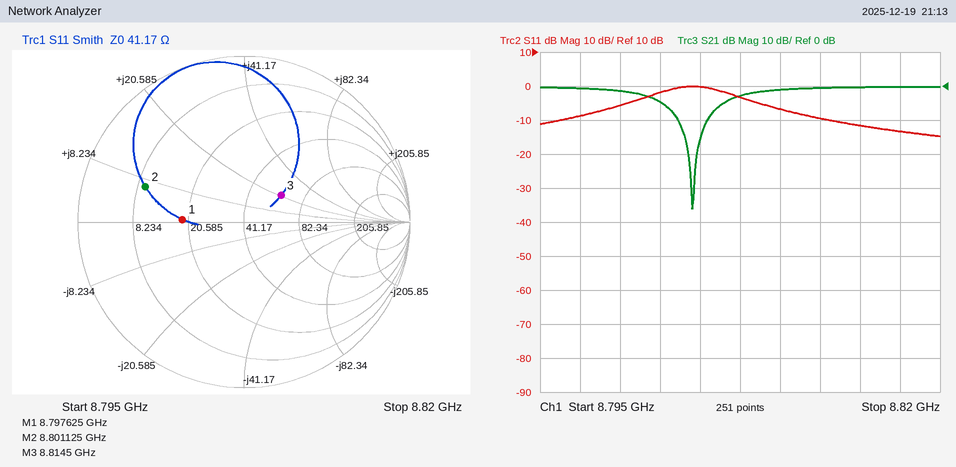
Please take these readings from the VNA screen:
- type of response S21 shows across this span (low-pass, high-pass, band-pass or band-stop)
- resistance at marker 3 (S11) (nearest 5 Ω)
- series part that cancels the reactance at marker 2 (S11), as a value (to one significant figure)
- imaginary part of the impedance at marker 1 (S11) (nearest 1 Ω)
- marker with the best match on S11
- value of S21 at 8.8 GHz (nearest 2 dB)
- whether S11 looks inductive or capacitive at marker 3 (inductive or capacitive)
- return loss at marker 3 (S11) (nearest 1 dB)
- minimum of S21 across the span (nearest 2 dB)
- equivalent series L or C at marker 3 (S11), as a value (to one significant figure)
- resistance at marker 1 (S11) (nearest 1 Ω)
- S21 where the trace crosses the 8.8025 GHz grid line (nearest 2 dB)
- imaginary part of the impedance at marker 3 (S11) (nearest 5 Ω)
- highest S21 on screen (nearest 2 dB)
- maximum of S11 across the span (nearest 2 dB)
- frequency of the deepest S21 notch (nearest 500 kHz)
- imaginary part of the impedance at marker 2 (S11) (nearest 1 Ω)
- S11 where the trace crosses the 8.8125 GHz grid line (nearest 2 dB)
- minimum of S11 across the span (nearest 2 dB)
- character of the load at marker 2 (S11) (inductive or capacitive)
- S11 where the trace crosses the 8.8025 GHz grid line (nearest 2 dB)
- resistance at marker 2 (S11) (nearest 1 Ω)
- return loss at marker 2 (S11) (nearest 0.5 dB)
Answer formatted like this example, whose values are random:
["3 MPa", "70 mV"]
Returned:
["band-stop", "60 Ω", "3 pF", "+1 Ω", "marker 3", "-2 dB", "inductive", "11 dB", "-36 dB", "400 pH", "19 Ω", "-4 dB", "+20 Ω", "0 dB", "0 dB", "8.8045 GHz", "+7 Ω", "-10 dB", "-14 dB", "inductive", "-2 dB", "10 Ω", "4.0 dB"]
